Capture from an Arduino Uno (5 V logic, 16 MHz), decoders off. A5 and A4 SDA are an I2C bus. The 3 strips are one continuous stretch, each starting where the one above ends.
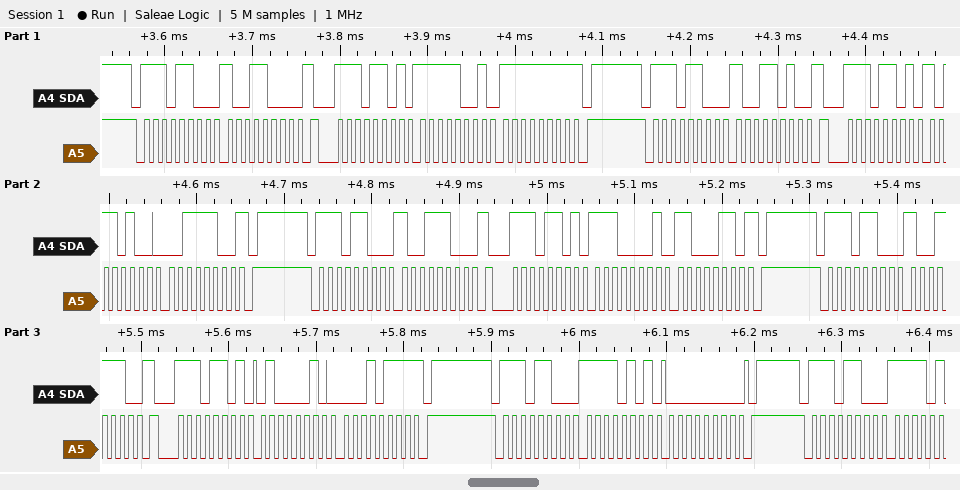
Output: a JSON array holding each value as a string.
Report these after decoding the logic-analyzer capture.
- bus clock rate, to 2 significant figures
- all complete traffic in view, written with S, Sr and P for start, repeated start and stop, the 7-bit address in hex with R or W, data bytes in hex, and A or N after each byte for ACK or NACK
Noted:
["100 kHz", "S 76W A 98 A Sr 76R A F9 A FF N P S 76W A 9A A Sr 76R A B4 A 3C N P S 76W A 9C A Sr 76R A E1 A C6 N P S 76W A 9E A Sr 76R A 42 A 17 N P S 76W A F5 A 00 A P S 76W A"]
